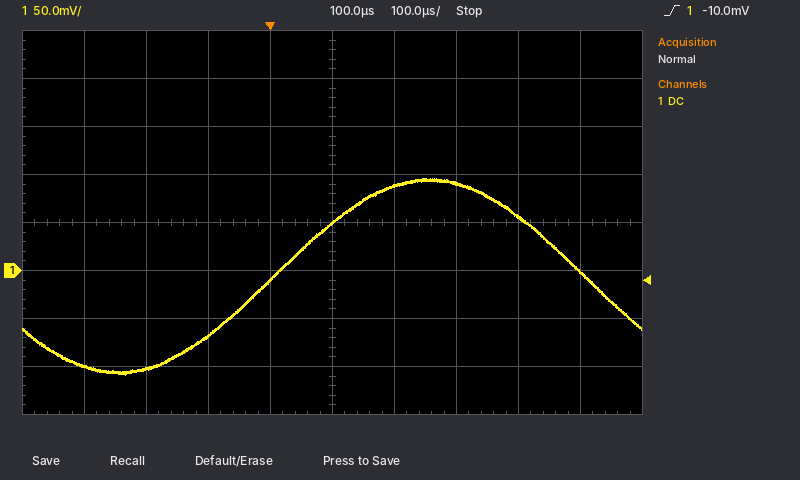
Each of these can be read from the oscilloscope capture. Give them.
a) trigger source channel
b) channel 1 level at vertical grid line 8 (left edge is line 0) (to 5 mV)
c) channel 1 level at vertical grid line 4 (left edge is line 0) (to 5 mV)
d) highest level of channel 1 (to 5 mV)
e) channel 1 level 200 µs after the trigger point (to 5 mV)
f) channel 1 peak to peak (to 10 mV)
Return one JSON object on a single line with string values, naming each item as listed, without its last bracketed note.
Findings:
{"trigger source channel": "channel 1", "channel 1 level at vertical grid line 8 (left edge is line 0)": "55 mV", "channel 1 level at vertical grid line 4 (left edge is line 0)": "-10 mV", "highest level of channel 1": "95 mV", "channel 1 level 200 µs after the trigger point": "90 mV", "channel 1 peak to peak": "200 mV"}
